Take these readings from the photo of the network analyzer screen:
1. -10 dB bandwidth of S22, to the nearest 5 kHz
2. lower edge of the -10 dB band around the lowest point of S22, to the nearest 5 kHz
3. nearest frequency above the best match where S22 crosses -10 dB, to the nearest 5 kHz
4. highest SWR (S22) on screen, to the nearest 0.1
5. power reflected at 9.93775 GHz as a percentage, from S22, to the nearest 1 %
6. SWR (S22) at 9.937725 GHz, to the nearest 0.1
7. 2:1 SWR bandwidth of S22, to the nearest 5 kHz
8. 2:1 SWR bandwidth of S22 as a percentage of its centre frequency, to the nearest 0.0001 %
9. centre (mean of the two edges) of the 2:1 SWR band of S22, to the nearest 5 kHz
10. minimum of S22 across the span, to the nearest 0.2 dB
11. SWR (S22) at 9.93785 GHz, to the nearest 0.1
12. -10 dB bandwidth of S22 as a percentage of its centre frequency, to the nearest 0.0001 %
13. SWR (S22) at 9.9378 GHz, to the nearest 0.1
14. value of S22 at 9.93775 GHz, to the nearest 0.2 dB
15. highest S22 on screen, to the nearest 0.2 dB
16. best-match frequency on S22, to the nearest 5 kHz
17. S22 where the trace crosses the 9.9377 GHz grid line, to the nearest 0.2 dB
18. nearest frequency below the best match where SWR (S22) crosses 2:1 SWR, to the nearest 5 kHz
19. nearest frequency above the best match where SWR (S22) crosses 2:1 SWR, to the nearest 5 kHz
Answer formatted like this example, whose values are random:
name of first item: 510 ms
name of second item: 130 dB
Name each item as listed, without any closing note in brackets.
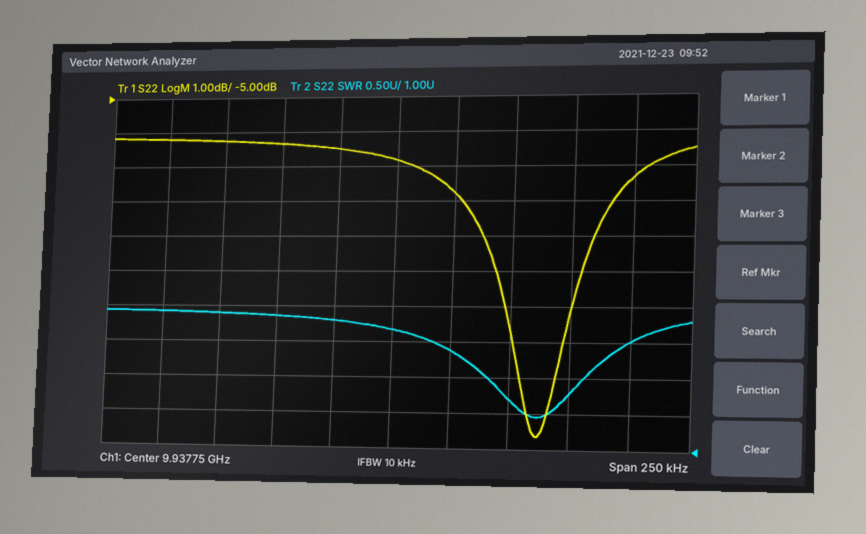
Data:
-10 dB bandwidth of S22, to the nearest 5 kHz: 35 kHz
lower edge of the -10 dB band around the lowest point of S22, to the nearest 5 kHz: 9.937795 GHz
nearest frequency above the best match where S22 crosses -10 dB, to the nearest 5 kHz: 9.937830 GHz
highest SWR (S22) on screen, to the nearest 0.1: 2.9
power reflected at 9.93775 GHz as a percentage, from S22, to the nearest 1 %: 21 %
SWR (S22) at 9.937725 GHz, to the nearest 0.1: 2.8
2:1 SWR bandwidth of S22, to the nearest 5 kHz: 40 kHz
2:1 SWR bandwidth of S22 as a percentage of its centre frequency, to the nearest 0.0001 %: 0.0004 %
centre (mean of the two edges) of the 2:1 SWR band of S22, to the nearest 5 kHz: 9.937810 GHz
minimum of S22 across the span, to the nearest 0.2 dB: -14.6 dB
SWR (S22) at 9.93785 GHz, to the nearest 0.1: 2.5
-10 dB bandwidth of S22 as a percentage of its centre frequency, to the nearest 0.0001 %: 0.0004 %
SWR (S22) at 9.9378 GHz, to the nearest 0.1: 1.7
value of S22 at 9.93775 GHz, to the nearest 0.2 dB: -6.8 dB
highest S22 on screen, to the nearest 0.2 dB: -6.2 dB
best-match frequency on S22, to the nearest 5 kHz: 9.937810 GHz
S22 where the trace crosses the 9.9377 GHz grid line, to the nearest 0.2 dB: -6.4 dB
nearest frequency below the best match where SWR (S22) crosses 2:1 SWR, to the nearest 5 kHz: 9.937790 GHz
nearest frequency above the best match where SWR (S22) crosses 2:1 SWR, to the nearest 5 kHz: 9.937830 GHz
